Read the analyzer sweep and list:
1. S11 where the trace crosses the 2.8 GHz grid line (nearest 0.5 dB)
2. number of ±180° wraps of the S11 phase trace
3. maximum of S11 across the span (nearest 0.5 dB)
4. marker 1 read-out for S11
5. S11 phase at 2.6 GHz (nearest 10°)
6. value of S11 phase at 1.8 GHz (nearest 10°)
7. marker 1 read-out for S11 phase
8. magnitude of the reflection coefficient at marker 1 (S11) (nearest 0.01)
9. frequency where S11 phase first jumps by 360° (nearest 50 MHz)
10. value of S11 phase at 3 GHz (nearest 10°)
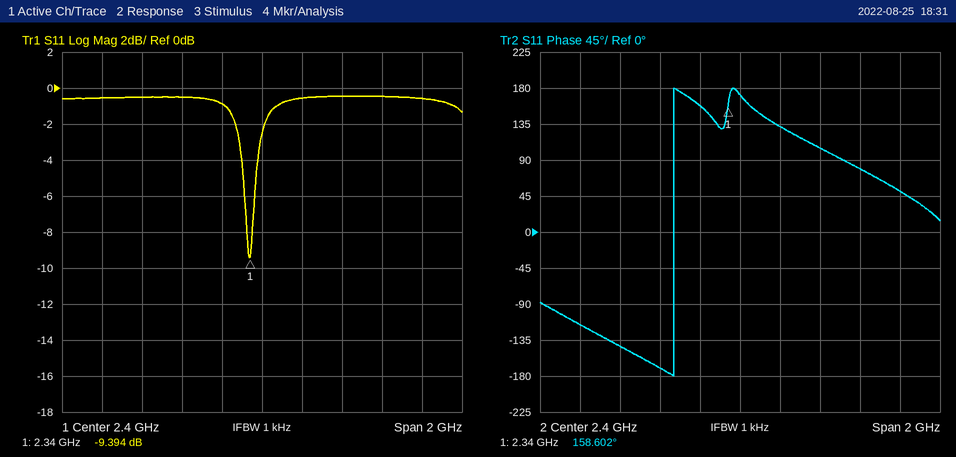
-0.5 dB
1
-0.5 dB
-9.394 dB
130°
-140°
158.602°
0.34
2.05 GHz
80°
